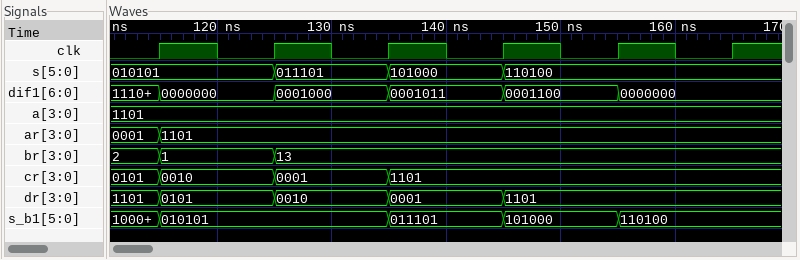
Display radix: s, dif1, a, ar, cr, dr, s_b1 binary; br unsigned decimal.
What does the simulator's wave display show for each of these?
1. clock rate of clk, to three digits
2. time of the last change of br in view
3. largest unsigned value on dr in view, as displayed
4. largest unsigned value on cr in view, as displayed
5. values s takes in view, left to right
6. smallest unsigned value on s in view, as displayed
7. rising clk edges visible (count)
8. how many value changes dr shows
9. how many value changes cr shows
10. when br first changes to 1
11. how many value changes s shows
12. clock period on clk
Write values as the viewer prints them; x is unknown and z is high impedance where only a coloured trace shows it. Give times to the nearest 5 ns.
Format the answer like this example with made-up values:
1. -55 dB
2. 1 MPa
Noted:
1. 100 MHz
2. 125 ns
3. 1101
4. 1101
5. 010101, 011101, 101000, 110100
6. 010101
7. 6
8. 4
9. 3
10. 115 ns
11. 3
12. 10 ns
